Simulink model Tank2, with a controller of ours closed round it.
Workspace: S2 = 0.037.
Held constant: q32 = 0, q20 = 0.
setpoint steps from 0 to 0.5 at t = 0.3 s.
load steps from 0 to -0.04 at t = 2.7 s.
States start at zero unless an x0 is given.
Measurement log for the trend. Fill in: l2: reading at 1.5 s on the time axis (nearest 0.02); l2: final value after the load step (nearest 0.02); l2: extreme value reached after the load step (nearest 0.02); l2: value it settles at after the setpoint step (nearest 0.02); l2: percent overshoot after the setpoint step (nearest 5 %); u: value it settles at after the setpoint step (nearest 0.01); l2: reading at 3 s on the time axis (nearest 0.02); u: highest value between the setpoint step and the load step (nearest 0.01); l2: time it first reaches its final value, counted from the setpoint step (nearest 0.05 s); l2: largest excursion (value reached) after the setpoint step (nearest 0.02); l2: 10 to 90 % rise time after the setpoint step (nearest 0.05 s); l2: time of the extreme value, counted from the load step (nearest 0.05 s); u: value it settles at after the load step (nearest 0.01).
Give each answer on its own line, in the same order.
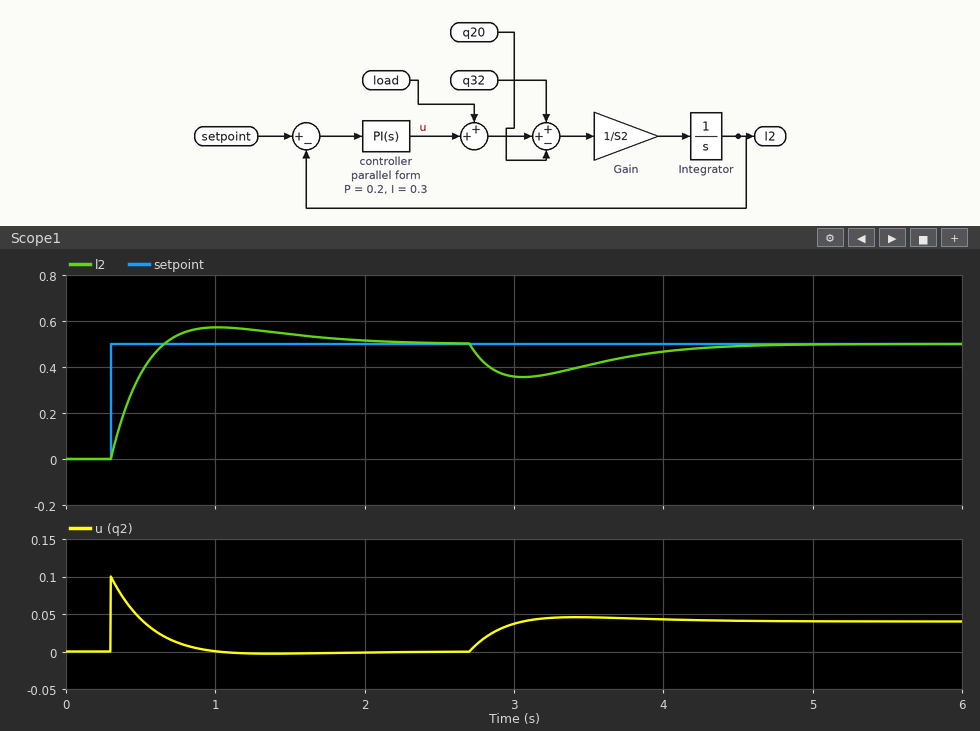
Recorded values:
0.54
0.50
0.36
0.50
15 %
0.00
0.36
0.10
0.35 s
0.58
0.25 s
0.35 s
0.04
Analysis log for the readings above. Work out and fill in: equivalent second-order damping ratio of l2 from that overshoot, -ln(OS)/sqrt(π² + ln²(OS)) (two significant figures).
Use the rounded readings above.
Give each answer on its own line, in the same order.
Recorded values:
0.52
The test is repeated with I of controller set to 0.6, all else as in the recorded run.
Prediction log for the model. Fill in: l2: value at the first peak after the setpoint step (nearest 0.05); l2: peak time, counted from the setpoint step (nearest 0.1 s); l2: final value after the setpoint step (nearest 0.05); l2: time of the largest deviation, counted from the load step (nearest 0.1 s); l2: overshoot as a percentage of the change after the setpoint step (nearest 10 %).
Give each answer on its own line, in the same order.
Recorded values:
0.60
0.6 s
0.50
0.3 s
20 %
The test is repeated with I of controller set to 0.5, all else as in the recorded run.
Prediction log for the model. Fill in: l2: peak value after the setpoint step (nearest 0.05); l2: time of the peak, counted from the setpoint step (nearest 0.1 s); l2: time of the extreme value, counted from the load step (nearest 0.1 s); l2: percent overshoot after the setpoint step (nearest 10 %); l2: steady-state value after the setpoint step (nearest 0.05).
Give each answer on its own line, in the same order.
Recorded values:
0.60
0.6 s
0.3 s
20 %
0.50
